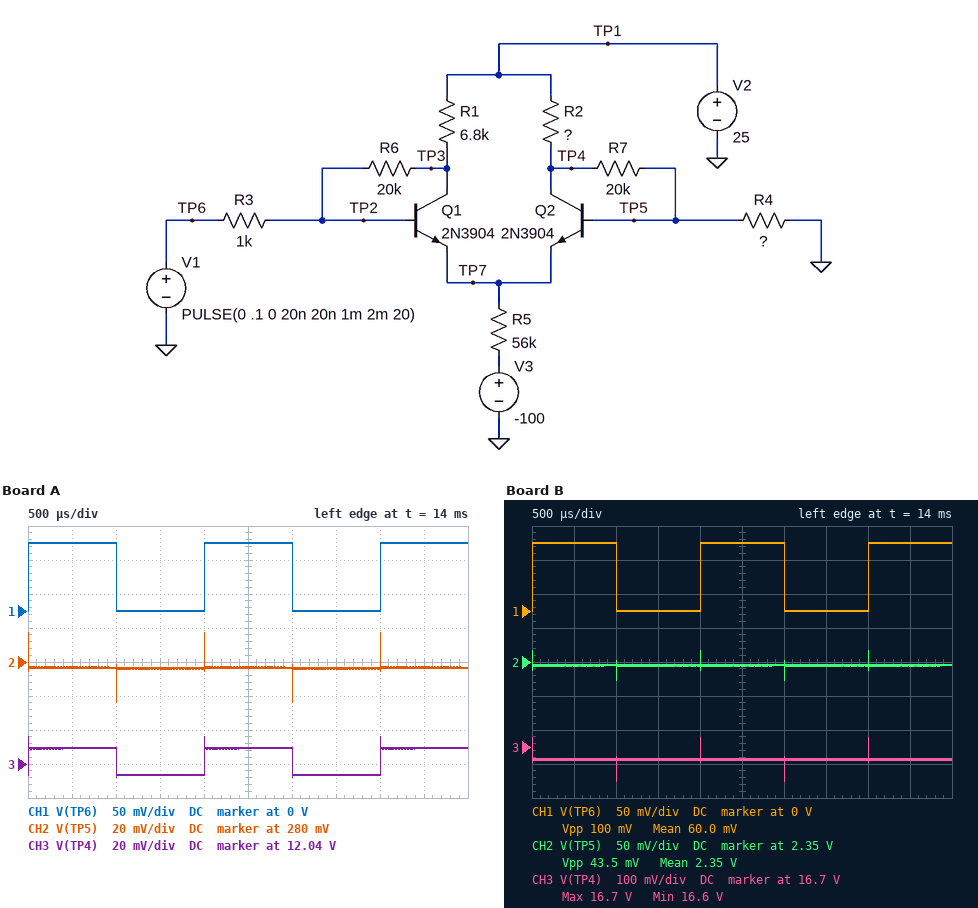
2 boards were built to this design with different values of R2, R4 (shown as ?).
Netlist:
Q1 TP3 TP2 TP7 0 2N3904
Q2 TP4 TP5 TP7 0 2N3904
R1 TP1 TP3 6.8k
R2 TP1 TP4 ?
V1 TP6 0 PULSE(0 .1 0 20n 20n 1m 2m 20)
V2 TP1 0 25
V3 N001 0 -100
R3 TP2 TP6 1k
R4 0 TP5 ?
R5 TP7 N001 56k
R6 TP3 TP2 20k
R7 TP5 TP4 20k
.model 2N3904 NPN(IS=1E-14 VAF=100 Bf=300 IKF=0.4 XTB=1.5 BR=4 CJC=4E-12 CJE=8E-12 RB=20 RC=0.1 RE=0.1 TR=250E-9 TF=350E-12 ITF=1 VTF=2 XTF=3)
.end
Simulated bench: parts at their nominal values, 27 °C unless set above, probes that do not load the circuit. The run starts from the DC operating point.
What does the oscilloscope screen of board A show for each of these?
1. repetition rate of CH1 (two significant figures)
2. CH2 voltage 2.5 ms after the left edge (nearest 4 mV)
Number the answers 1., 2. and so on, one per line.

1. 500 Hz
2. 276 mV
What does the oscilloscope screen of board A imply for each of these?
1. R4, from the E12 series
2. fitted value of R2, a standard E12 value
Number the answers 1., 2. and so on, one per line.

1. 470 Ω
2. 22 kΩ
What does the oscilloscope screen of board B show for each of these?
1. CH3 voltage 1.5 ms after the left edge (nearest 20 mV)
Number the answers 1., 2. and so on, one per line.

1. 16.66 V
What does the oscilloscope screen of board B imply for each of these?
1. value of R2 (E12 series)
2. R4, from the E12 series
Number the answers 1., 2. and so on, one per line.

1. 3.3 kΩ
2. 3.3 kΩ
